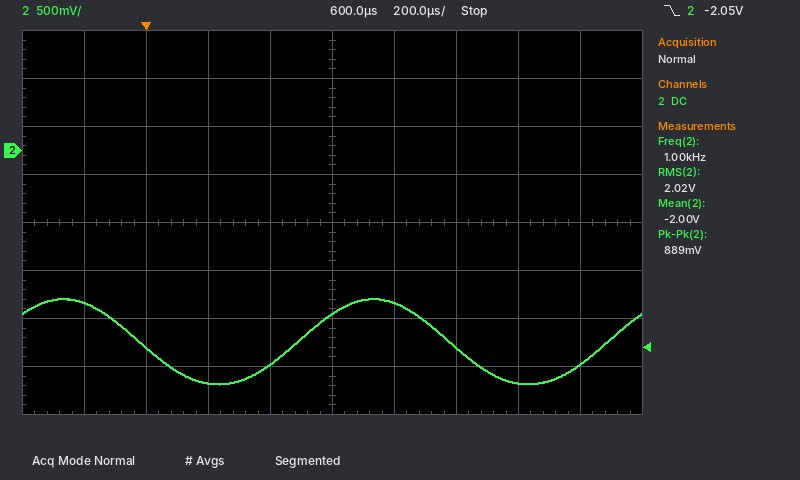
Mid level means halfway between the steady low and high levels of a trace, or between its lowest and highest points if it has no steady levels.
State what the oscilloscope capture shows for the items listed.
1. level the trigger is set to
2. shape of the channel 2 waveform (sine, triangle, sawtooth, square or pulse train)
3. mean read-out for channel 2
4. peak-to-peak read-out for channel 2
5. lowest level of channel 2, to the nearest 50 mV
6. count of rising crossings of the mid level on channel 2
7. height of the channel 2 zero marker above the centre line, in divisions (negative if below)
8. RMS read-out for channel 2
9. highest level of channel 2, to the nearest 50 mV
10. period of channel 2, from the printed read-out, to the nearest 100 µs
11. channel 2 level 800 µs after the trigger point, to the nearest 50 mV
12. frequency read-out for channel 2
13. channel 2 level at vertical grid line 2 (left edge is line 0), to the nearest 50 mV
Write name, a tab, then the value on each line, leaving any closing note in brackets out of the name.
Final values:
level the trigger is set to	-2.05 V
shape of the channel 2 waveform	sine
mean read-out for channel 2	-2.00 V
peak-to-peak read-out for channel 2	889 mV
lowest level of channel 2, to the nearest 50 mV	-2.45 V
count of rising crossings of the mid level on channel 2	2
height of the channel 2 zero marker above the centre line, in divisions	+1.5 div
RMS read-out for channel 2	2.02 V
highest level of channel 2, to the nearest 50 mV	-1.55 V
period of channel 2, from the printed read-out, to the nearest 100 µs	1.0 ms
channel 2 level 800 µs after the trigger point, to the nearest 50 mV	-1.60 V
frequency read-out for channel 2	1.00 kHz
channel 2 level at vertical grid line 2 (left edge is line 0), to the nearest 50 mV	-2.05 V
